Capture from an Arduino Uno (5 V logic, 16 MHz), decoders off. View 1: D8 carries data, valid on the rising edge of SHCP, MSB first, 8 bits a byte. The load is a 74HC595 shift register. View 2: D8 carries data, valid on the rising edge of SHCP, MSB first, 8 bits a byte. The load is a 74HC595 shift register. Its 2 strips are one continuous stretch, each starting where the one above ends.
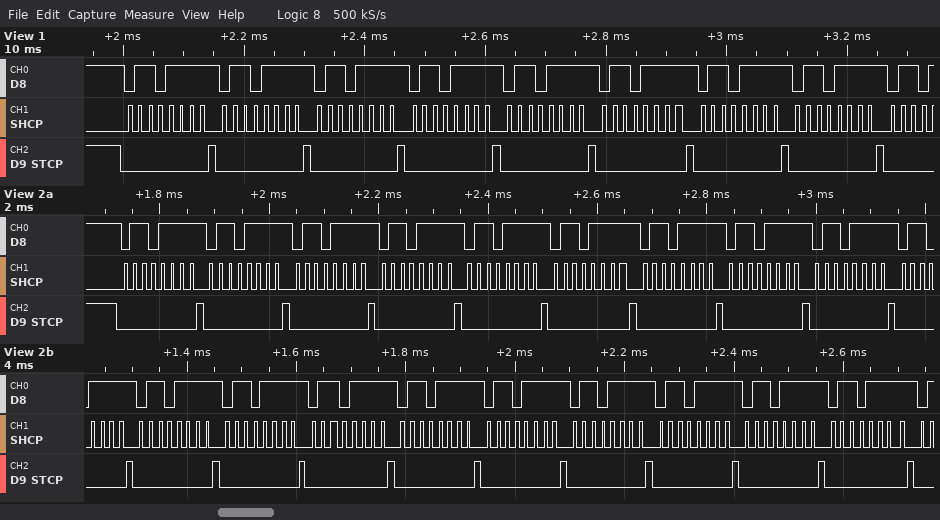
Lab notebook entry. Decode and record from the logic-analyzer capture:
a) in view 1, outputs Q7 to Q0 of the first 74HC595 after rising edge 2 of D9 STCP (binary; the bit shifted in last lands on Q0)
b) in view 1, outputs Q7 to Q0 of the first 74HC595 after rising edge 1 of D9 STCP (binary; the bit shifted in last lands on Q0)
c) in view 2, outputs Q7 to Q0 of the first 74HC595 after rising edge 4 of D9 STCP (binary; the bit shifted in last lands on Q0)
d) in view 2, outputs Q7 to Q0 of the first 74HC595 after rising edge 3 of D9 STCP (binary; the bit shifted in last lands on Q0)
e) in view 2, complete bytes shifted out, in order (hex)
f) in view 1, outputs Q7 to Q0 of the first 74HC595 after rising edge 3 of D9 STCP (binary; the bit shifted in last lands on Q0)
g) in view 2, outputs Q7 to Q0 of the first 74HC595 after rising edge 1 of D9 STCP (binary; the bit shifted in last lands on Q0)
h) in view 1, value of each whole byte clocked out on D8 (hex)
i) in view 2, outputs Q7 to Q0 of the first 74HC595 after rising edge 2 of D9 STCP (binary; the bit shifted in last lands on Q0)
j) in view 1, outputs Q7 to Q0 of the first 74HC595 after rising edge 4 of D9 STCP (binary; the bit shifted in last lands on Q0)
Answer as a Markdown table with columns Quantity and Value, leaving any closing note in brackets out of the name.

| Quantity | Value |
|---|---|
| in view 1, outputs Q7 to Q0 of the first 74HC595 after rising edge 2 of D9 STCP | 01101111 |
| in view 1, outputs Q7 to Q0 of the first 74HC595 after rising edge 1 of D9 STCP | 01101111 |
| in view 2, outputs Q7 to Q0 of the first 74HC595 after rising edge 4 of D9 STCP | 01101111 |
| in view 2, outputs Q7 to Q0 of the first 74HC595 after rising edge 3 of D9 STCP | 01101111 |
| in view 2, complete bytes shifted out, in order | 6F 6F 6F 6F 6F 6F 6F 6F 6F 6F 6F 6F 6F 6F 6F 6F 6F 6F 6F |
| in view 1, outputs Q7 to Q0 of the first 74HC595 after rising edge 3 of D9 STCP | 01101111 |
| in view 2, outputs Q7 to Q0 of the first 74HC595 after rising edge 1 of D9 STCP | 01101111 |
| in view 1, value of each whole byte clocked out on D8 | 6F 6F 6F 6F 6F 6F 6F 6F |
| in view 2, outputs Q7 to Q0 of the first 74HC595 after rising edge 2 of D9 STCP | 01101111 |
| in view 1, outputs Q7 to Q0 of the first 74HC595 after rising edge 4 of D9 STCP | 01101111 |
